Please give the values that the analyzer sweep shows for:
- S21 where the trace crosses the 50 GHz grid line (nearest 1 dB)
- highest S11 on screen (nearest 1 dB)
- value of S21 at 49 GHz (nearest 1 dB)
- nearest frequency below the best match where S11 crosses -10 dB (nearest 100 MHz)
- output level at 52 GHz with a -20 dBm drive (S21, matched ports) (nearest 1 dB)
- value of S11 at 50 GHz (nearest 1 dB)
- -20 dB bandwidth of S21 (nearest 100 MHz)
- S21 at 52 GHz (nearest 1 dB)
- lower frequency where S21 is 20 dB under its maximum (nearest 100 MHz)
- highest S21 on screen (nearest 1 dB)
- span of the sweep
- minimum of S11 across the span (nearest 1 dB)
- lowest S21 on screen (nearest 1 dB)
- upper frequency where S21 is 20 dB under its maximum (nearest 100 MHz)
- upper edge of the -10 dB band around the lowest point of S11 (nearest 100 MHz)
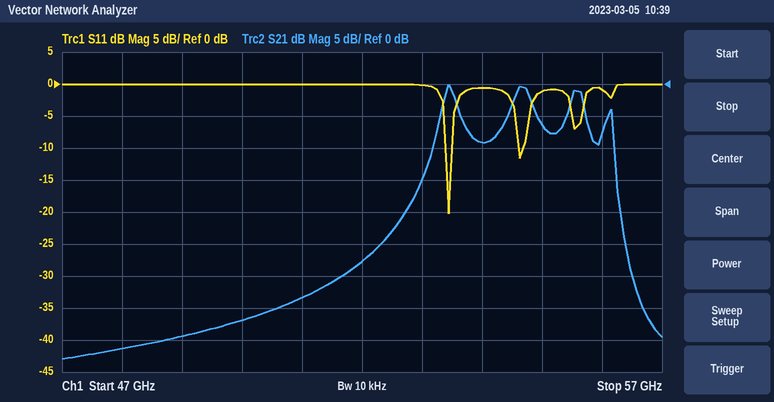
-37 dB
0 dB
-39 dB
53.4 GHz
-48 dBm
0 dB
3.6 GHz
-28 dB
52.7 GHz
0 dB
10 GHz
-20 dB
-43 dB
56.3 GHz
53.5 GHz
